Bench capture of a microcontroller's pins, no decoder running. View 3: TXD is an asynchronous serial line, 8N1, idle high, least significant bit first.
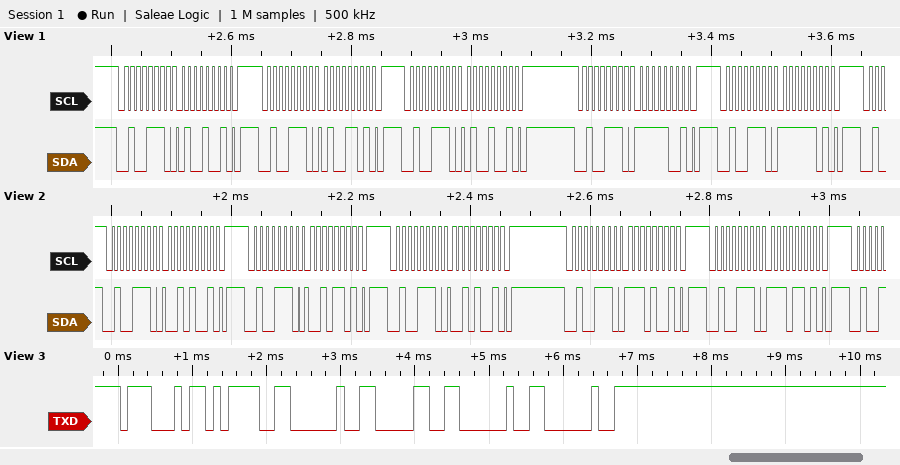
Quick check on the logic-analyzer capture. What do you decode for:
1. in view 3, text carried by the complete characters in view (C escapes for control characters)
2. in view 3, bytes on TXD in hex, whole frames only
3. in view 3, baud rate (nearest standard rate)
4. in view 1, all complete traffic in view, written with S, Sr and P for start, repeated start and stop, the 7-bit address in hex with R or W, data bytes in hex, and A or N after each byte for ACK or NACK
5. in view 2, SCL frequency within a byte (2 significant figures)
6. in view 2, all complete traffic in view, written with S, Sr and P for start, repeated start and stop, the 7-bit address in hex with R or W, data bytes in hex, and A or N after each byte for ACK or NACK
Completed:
"G= 0  "
0x47 0x3D 0x20 0x30 0x20 0x20
9600 baud
S 27W A 49 A P S 27W A 4D A P S 27W A 49 A P S 27W A F9 A P S 27W A FD A P
100 kHz
S 27W A 29 A P S 27W A 2D A P S 27W A 29 A P S 27W A E9 A P S 27W A ED A P
